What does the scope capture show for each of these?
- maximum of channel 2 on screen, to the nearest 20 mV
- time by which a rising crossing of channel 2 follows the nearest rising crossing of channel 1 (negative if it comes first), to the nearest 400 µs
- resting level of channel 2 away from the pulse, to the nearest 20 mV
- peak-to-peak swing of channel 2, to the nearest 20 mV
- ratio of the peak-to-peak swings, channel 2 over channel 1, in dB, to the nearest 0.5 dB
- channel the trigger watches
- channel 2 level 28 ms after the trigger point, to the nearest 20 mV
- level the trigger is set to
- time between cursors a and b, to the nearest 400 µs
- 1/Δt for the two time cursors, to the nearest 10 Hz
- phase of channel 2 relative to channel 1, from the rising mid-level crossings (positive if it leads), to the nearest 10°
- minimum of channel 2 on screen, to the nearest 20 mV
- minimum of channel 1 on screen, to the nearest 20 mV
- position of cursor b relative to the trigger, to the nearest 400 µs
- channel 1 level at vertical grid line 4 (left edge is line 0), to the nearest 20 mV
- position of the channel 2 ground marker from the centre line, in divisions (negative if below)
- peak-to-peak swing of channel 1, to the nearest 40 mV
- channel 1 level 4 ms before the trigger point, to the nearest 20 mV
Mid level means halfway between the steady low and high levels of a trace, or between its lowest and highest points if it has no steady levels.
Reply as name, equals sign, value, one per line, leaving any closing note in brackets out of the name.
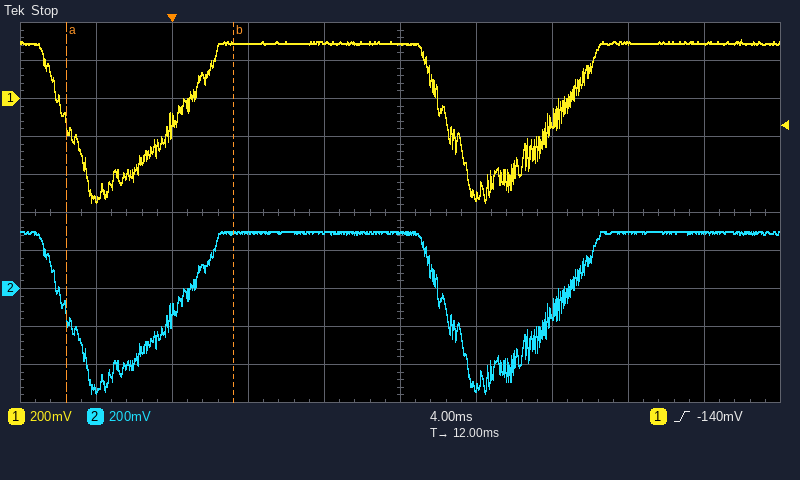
maximum of channel 2 on screen, to the nearest 20 mV = 300 mV
time by which a rising crossing of channel 2 follows the nearest rising crossing of channel 1 (negative if it comes first), to the nearest 400 µs = 0.0 ms
resting level of channel 2 away from the pulse, to the nearest 20 mV = 300 mV
peak-to-peak swing of channel 2, to the nearest 20 mV = 860 mV
ratio of the peak-to-peak swings, channel 2 over channel 1, in dB, to the nearest 0.5 dB = 0.0 dB
channel the trigger watches = channel 1
channel 2 level 28 ms after the trigger point, to the nearest 20 mV = 300 mV
level the trigger is set to = -140 mV
time between cursors a and b, to the nearest 400 µs = 8.8 ms
1/Δt for the two time cursors, to the nearest 10 Hz = 110 Hz
phase of channel 2 relative to channel 1, from the rising mid-level crossings (positive if it leads), to the nearest 10° = 0°
minimum of channel 2 on screen, to the nearest 20 mV = -560 mV
minimum of channel 1 on screen, to the nearest 20 mV = -540 mV
position of cursor b relative to the trigger, to the nearest 400 µs = +3.2 ms
channel 1 level at vertical grid line 4 (left edge is line 0), to the nearest 20 mV = 300 mV
position of the channel 2 ground marker from the centre line, in divisions = -2.0 div
peak-to-peak swing of channel 1, to the nearest 40 mV = 840 mV
channel 1 level 4 ms before the trigger point, to the nearest 20 mV = -520 mV
